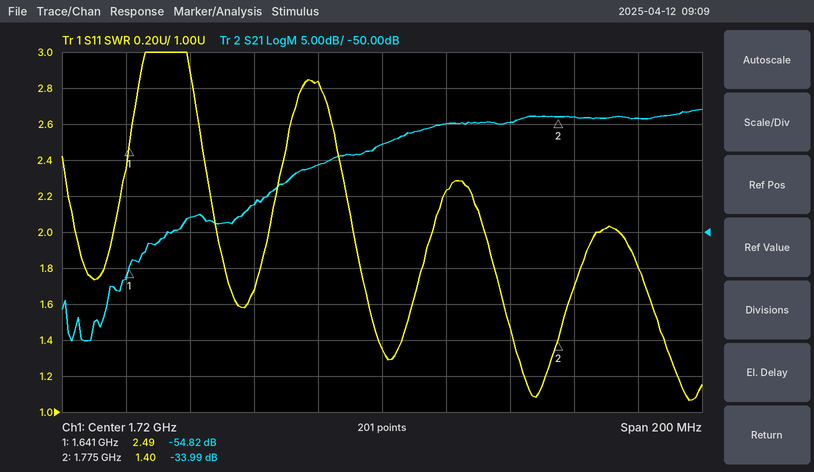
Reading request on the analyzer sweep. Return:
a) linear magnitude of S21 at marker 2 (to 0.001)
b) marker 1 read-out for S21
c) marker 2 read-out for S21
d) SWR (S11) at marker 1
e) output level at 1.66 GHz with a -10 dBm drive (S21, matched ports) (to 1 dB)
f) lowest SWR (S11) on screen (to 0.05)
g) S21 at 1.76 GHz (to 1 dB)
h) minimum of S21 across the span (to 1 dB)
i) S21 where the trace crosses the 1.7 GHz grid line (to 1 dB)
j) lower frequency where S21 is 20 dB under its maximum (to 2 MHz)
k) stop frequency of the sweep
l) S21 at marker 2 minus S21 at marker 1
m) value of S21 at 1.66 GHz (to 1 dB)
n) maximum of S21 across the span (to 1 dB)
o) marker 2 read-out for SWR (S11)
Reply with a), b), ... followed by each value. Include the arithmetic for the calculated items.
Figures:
a) 10^(-33.99/20) ≈ 0.020
b) -54.82 dB
c) -33.99 dB
d) 2.49
e) -10 dBm + (-48 dB) = -58 dBm
f) 1.05
g) -35 dB
h) -65 dB
i) -41 dB
j) 1.646 GHz
k) 1.82 GHz
l) -33.99 − (-54.82) = 20.83 dB
m) -48 dB
n) -33 dB
o) 1.40
